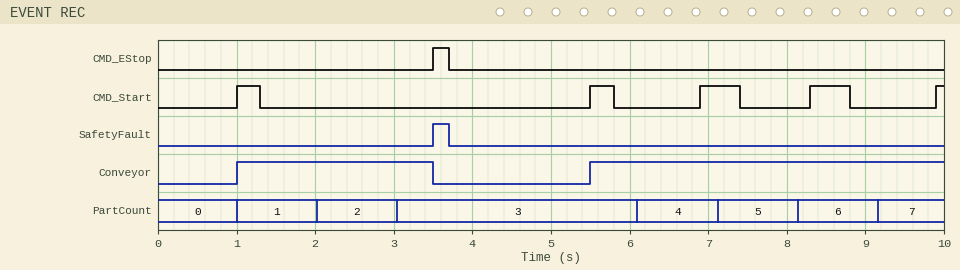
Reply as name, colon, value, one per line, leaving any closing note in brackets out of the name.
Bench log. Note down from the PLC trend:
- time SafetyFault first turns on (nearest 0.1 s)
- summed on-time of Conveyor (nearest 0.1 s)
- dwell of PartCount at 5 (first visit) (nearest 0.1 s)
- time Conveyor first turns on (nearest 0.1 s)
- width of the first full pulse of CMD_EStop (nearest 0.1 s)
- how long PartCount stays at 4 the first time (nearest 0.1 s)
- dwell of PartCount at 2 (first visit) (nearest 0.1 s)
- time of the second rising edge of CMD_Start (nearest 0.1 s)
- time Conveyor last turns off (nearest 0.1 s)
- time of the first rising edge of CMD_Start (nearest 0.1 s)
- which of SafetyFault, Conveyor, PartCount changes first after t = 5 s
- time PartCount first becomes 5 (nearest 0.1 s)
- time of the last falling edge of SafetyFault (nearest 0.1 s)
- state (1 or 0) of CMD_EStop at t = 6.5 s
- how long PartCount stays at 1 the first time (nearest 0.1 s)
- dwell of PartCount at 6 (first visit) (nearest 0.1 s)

time SafetyFault first turns on: 3.5 s
summed on-time of Conveyor: 7.0 s
dwell of PartCount at 5 (first visit): 1.0 s
time Conveyor first turns on: 1.0 s
width of the first full pulse of CMD_EStop: 0.2 s
how long PartCount stays at 4 the first time: 1.0 s
dwell of PartCount at 2 (first visit): 1.0 s
time of the second rising edge of CMD_Start: 5.5 s
time Conveyor last turns off: 3.5 s
time of the first rising edge of CMD_Start: 1.0 s
which of SafetyFault, Conveyor, PartCount changes first after t = 5 s: Conveyor
time PartCount first becomes 5: 7.1 s
time of the last falling edge of SafetyFault: 3.7 s
state (1 or 0) of CMD_EStop at t = 6.5 s: 0
how long PartCount stays at 1 the first time: 1.0 s
dwell of PartCount at 6 (first visit): 1.0 s
